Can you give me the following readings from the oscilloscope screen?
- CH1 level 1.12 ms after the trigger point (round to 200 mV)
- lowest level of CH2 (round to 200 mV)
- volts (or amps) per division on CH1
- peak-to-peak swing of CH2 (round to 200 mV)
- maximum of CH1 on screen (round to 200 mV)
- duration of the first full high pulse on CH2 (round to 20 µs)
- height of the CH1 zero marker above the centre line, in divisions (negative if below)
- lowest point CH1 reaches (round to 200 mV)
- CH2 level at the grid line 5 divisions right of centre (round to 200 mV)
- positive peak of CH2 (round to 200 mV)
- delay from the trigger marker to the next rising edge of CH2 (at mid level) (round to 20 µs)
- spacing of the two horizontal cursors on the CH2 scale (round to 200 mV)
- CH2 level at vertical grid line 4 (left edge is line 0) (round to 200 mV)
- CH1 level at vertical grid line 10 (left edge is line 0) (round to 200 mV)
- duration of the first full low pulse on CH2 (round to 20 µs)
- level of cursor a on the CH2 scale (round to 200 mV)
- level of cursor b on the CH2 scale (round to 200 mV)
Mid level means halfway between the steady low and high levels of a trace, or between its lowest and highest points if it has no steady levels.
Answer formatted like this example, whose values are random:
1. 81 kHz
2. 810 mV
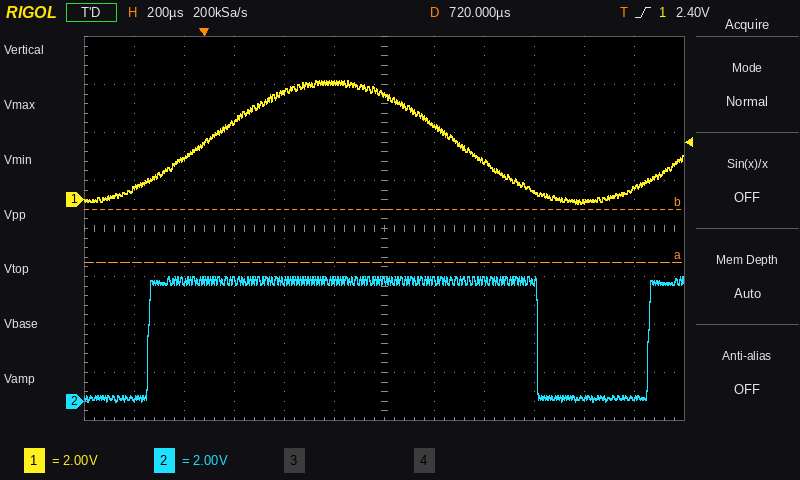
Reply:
1. 1.6 V
2. 0.0 V
3. 2 V
4. 5.2 V
5. 5.0 V
6. 1.56 ms
7. +0.6 div
8. -200 mV
9. 200 mV
10. 5.2 V
11. 1.78 ms
12. 2.2 V
13. 5.0 V
14. 0.0 V
15. 440 µs
16. 5.8 V
17. 8.0 V
